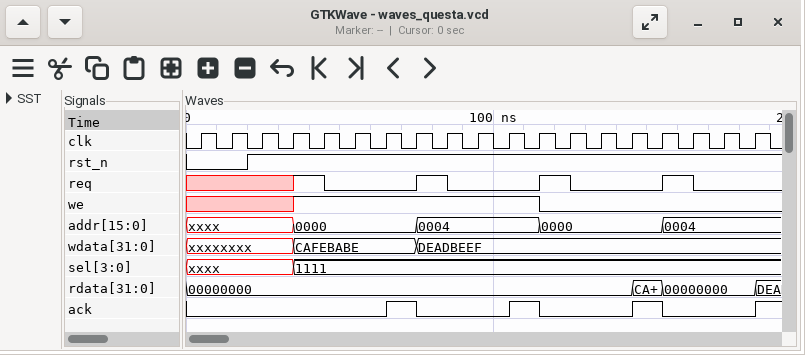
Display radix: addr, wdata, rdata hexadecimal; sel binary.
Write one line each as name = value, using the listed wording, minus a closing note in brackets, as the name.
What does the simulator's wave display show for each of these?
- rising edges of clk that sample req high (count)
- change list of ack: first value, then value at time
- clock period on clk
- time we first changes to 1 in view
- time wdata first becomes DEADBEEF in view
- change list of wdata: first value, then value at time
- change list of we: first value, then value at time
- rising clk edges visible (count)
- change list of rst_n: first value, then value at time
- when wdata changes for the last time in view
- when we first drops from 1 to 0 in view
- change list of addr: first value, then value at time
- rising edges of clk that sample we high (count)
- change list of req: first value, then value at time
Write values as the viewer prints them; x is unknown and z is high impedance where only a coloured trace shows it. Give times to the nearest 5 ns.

rising edges of clk that sample req high = 4
change list of ack: first value, then value at time = 0, 1 at 65 ns, 0 at 75 ns, 1 at 105 ns, 0 at 115 ns, 1 at 145 ns, 0 at 155 ns, 1 at 185 ns
clock period on clk = 10 ns
time we first changes to 1 in view = 35 ns
time wdata first becomes DEADBEEF in view = 75 ns
change list of wdata: first value, then value at time = xxxxxxxx, CAFEBABE at 35 ns, DEADBEEF at 75 ns
change list of we: first value, then value at time = x, 1 at 35 ns, 0 at 115 ns
rising clk edges visible = 19
change list of rst_n: first value, then value at time = 0, 1 at 20 ns
when wdata changes for the last time in view = 75 ns
when we first drops from 1 to 0 in view = 115 ns
change list of addr: first value, then value at time = xxxx, 0000 at 35 ns, 0004 at 75 ns, 0000 at 115 ns, 0004 at 155 ns
rising edges of clk that sample we high = 8
change list of req: first value, then value at time = x, 1 at 35 ns, 0 at 45 ns, 1 at 75 ns, 0 at 85 ns, 1 at 115 ns, 0 at 125 ns, 1 at 155 ns, 0 at 165 ns
